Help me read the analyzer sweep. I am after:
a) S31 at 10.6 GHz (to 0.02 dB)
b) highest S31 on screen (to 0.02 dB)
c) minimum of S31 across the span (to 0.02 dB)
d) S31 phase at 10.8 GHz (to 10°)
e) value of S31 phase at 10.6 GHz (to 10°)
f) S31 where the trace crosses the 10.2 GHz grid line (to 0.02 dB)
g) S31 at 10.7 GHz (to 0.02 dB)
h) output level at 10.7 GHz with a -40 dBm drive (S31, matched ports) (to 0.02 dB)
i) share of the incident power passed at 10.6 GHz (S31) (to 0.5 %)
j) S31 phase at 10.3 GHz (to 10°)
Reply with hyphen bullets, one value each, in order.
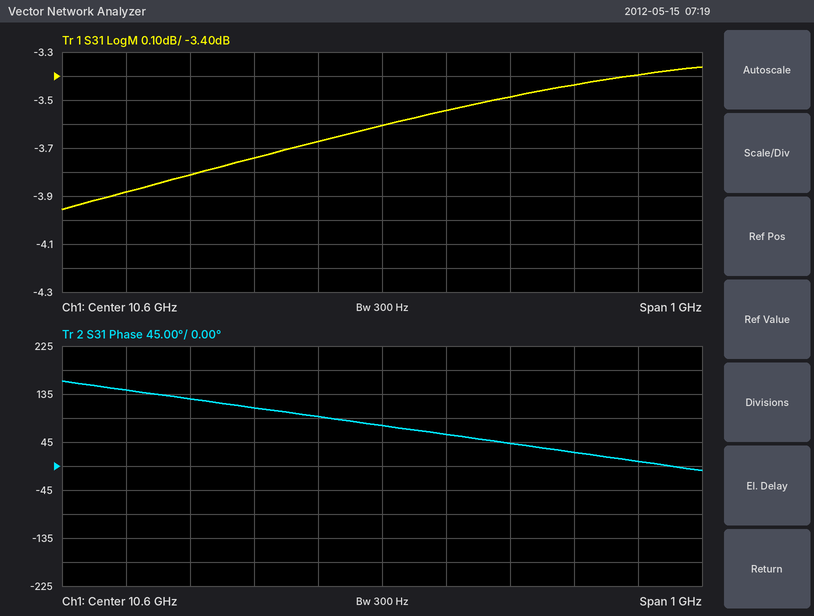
- -3.60 dB
- -3.36 dB
- -3.96 dB
- 40°
- 80°
- -3.88 dB
- -3.54 dB
- -43.54 dBm
- 43.5 %
- 130°
